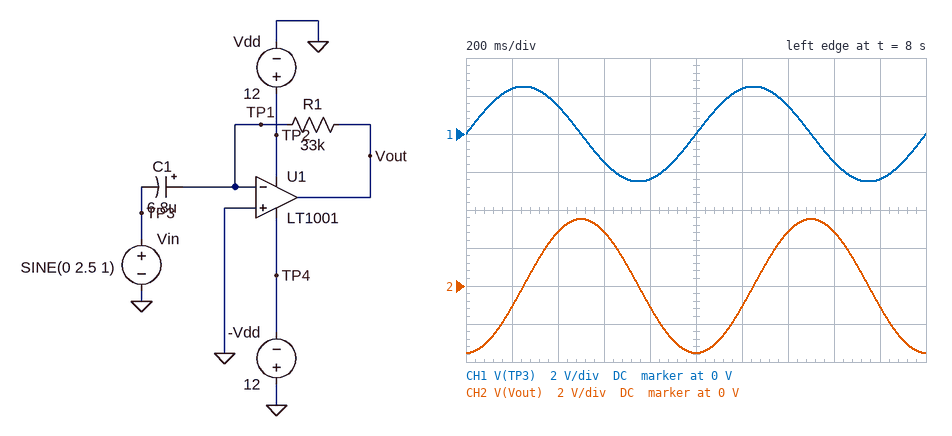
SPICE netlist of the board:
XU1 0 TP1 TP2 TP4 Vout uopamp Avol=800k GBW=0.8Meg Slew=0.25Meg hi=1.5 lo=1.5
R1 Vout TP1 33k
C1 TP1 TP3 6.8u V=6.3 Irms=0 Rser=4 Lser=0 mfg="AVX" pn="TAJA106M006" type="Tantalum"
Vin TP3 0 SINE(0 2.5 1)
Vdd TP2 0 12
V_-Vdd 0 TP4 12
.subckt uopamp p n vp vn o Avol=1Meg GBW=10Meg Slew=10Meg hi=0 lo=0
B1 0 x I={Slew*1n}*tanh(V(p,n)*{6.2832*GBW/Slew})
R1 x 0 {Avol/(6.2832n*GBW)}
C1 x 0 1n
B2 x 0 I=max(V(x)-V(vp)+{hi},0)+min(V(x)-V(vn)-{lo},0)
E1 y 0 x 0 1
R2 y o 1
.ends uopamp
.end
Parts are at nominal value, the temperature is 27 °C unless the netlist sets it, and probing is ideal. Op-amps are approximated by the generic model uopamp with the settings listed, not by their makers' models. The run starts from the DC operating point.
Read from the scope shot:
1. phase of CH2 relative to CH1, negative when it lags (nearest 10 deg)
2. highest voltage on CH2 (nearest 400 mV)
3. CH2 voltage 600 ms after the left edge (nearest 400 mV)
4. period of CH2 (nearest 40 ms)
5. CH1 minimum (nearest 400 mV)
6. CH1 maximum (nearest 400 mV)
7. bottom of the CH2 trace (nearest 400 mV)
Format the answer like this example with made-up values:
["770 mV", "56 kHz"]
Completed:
["-90 deg", "3.6 V", "2.8 V", "1.00 s", "-2.4 V", "2.4 V", "-3.6 V"]
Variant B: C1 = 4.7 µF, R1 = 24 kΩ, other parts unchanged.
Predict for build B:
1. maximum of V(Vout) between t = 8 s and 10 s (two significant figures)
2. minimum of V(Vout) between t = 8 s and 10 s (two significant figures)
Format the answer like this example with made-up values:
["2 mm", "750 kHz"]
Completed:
["1.8 V", "-1.8 V"]
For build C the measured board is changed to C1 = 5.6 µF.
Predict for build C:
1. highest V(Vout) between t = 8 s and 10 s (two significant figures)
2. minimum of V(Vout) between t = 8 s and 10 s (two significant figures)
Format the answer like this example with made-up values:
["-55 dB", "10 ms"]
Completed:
["2.9 V", "-2.9 V"]
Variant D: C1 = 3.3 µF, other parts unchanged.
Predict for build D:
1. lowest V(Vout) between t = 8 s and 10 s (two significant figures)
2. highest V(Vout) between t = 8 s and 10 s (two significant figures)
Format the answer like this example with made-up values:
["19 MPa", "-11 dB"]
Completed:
["-1.7 V", "1.7 V"]
